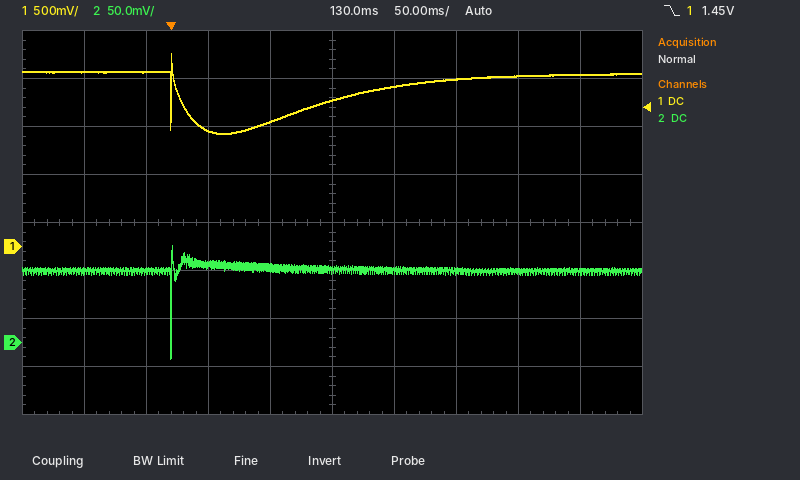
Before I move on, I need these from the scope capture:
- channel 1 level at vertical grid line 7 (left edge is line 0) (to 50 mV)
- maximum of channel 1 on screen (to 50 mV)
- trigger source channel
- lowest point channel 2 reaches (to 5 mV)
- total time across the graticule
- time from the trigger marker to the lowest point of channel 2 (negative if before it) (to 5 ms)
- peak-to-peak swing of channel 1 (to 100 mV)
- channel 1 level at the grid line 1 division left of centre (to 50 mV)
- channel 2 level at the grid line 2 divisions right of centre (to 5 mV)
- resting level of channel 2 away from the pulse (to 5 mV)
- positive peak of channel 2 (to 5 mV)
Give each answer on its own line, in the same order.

1.75 V
2.00 V
channel 1
-15 mV
500 ms
0 ms
800 mV
1.30 V
75 mV
75 mV
100 mV
